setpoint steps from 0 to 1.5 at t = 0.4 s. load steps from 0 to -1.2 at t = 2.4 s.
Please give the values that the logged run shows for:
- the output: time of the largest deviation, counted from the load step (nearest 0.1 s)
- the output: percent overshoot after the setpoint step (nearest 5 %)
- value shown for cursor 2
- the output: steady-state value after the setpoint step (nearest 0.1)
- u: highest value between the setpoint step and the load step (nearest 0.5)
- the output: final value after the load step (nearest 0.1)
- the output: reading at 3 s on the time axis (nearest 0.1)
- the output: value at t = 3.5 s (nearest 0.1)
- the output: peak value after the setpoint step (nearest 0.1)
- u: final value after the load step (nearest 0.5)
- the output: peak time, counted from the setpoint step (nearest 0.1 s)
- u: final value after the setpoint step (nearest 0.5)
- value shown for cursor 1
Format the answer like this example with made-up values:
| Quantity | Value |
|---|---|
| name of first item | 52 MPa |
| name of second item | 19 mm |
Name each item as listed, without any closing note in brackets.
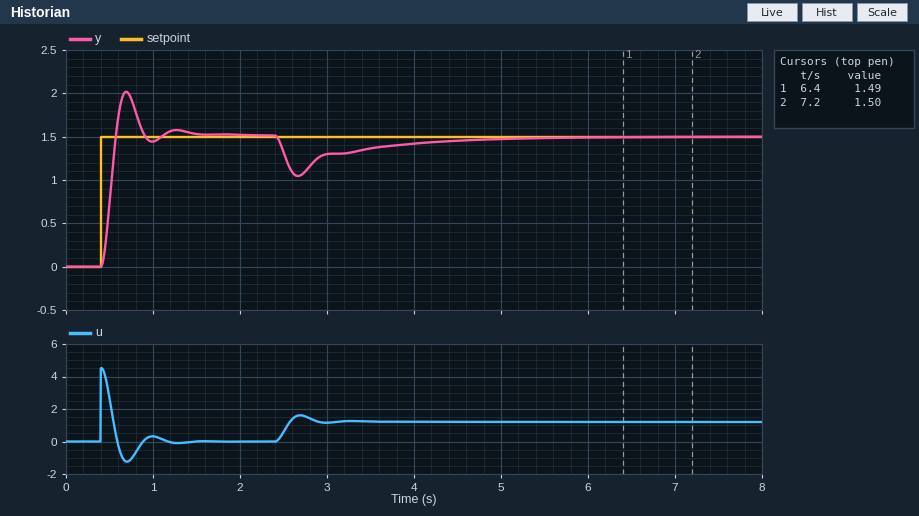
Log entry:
| Quantity | Value |
|---|---|
| the output: time of the largest deviation, counted from the load step | 0.3 s |
| the output: percent overshoot after the setpoint step | 35 % |
| value shown for cursor 2 | 1.50 |
| the output: steady-state value after the setpoint step | 1.5 |
| u: highest value between the setpoint step and the load step | 4.5 |
| the output: final value after the load step | 1.5 |
| the output: reading at 3 s on the time axis | 1.3 |
| the output: value at t = 3.5 s | 1.4 |
| the output: peak value after the setpoint step | 2.0 |
| u: final value after the load step | 1.0 |
| the output: peak time, counted from the setpoint step | 0.3 s |
| u: final value after the setpoint step | 0.0 |
| value shown for cursor 1 | 1.49 |
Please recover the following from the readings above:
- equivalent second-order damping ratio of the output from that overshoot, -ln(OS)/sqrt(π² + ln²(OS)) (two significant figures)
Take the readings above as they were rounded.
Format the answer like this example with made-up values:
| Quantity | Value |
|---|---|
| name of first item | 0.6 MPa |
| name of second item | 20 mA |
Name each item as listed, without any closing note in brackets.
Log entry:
| Quantity | Value |
|---|---|
| equivalent second-order damping ratio of the output from that overshoot, -ln(OS)/sqrt(π² + ln²(OS)) | 0.32 |
